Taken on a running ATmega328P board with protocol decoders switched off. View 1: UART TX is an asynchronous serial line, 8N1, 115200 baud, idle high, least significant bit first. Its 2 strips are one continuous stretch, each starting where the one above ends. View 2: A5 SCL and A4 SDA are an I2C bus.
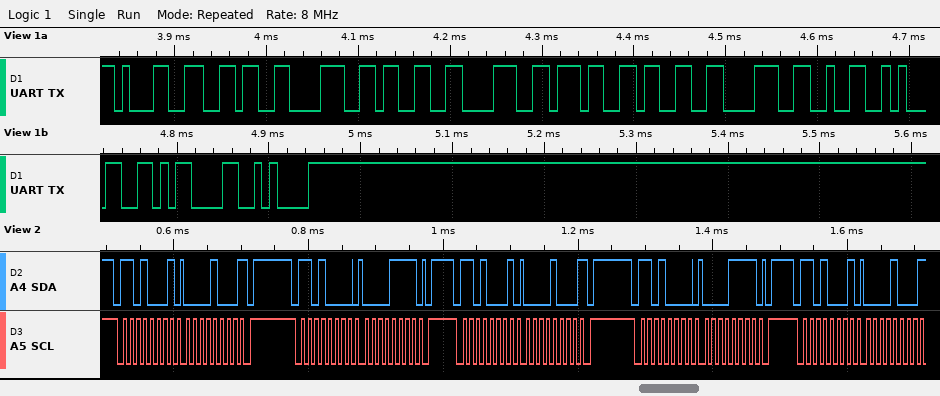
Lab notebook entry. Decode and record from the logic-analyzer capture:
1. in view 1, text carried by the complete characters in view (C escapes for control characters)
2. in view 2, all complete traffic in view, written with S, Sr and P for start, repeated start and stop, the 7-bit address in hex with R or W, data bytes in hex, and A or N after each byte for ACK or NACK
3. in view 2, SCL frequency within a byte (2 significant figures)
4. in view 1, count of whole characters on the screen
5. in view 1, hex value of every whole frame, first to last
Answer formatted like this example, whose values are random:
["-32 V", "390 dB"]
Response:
["\"1683873821\\r\\n\"", "S 68R A 08 N P S 68W A 0F A P S 68R A 08 N P S 68W A 0F A P S 68R A 08 N", "100 kHz", "12", "31 36 38 33 38 37 33 38 32 31 0D 0A"]
